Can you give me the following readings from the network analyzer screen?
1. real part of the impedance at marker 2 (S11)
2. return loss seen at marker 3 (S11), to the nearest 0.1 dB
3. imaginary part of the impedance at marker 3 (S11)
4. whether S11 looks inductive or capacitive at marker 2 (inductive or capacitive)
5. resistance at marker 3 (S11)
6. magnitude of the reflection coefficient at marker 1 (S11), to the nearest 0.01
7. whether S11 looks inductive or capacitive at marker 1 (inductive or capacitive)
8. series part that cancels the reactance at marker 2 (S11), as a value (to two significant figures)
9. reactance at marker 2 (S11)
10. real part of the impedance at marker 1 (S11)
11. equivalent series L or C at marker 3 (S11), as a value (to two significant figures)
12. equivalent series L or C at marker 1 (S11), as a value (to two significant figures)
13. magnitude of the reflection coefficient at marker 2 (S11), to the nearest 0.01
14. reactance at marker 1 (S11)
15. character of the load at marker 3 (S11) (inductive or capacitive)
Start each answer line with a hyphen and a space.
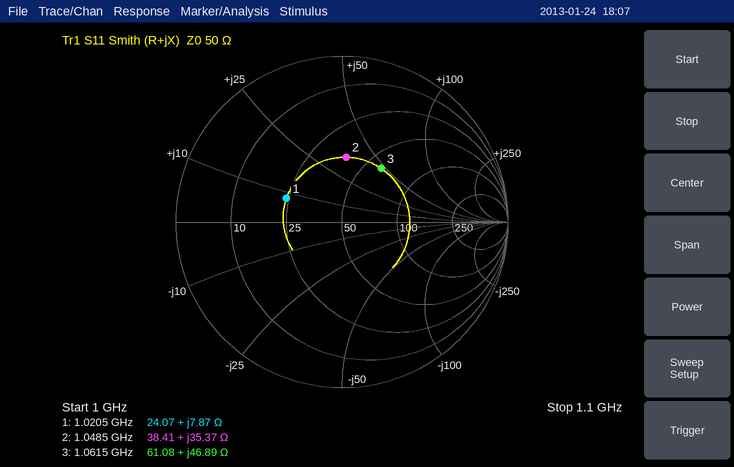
- 38.41 Ω
- 8.0 dB
- +46.89 Ω
- inductive
- 61.08 Ω
- 0.36
- inductive
- 4.3 pF
- +35.37 Ω
- 24.07 Ω
- 7.0 nH
- 1.2 nH
- 0.39
- +7.87 Ω
- inductive
